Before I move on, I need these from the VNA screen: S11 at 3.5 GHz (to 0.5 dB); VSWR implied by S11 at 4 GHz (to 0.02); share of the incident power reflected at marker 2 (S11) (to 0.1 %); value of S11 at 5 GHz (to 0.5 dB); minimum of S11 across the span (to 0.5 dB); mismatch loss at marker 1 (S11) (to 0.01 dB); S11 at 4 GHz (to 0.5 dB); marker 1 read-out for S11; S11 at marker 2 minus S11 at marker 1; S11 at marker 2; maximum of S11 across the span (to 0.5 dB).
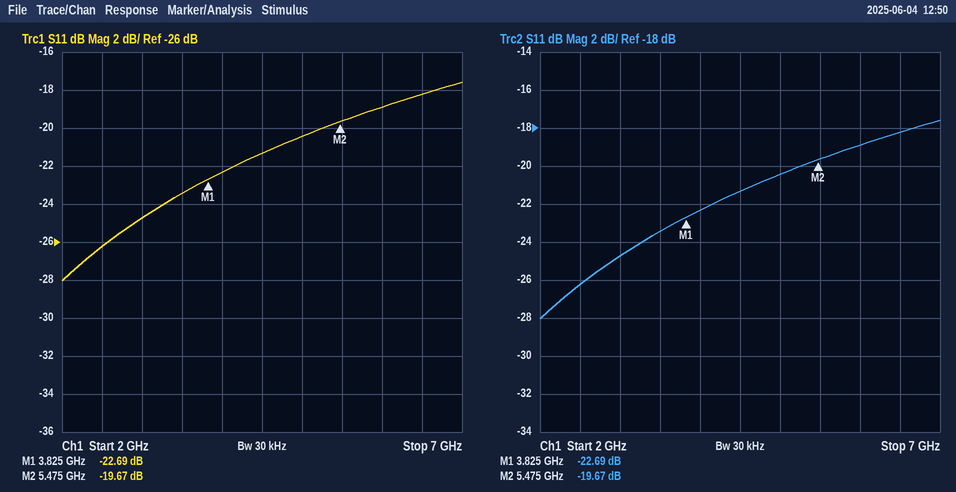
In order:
-23.5 dB
1.16
1.1 %
-20.5 dB
-28.0 dB
0.02 dB
-22.5 dB
-22.69 dB
3.02 dB
-19.67 dB
-17.5 dB
